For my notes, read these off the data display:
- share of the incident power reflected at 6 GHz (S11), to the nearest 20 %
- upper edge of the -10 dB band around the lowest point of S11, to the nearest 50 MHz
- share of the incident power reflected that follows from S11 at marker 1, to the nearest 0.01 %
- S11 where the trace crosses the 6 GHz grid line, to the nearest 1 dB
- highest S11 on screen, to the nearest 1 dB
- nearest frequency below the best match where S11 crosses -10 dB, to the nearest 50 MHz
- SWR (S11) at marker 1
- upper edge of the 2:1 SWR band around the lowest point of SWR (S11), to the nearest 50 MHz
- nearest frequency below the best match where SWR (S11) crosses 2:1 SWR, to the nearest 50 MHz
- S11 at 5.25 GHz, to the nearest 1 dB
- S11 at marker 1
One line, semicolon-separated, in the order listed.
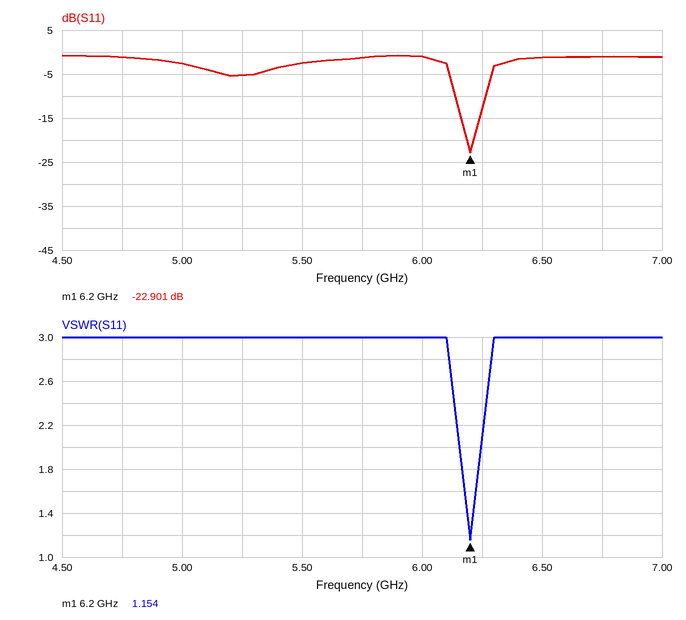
80 %; 6.25 GHz; 0.51 %; -1 dB; -1 dB; 6.15 GHz; 1.154; 6.25 GHz; 6.15 GHz; -5 dB; -22.901 dB
